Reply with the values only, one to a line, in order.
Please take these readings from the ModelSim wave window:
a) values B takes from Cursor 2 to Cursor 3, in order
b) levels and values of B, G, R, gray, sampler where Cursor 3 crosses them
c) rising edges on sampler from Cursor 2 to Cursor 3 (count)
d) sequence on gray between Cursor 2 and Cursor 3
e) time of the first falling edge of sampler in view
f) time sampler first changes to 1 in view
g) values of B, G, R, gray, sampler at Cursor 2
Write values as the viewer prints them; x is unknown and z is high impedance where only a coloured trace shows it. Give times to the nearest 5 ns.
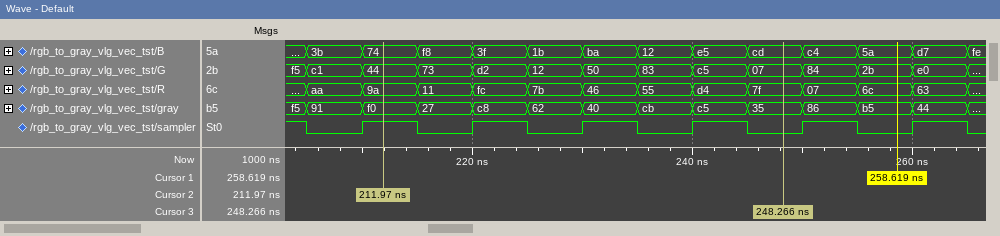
74, f8, 3f, 1b, ba, 12, e5, cd
B=cd, G=07, R=7f, gray=35, sampler=0
3
f0, 27, c8, 62, 40, cb, c5, 35
205 ns
210 ns
B=74, G=44, R=9a, gray=f0, sampler=1
